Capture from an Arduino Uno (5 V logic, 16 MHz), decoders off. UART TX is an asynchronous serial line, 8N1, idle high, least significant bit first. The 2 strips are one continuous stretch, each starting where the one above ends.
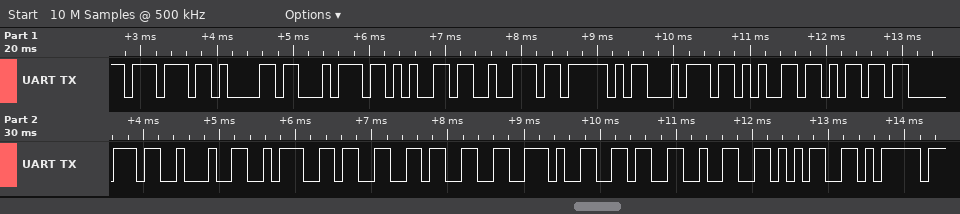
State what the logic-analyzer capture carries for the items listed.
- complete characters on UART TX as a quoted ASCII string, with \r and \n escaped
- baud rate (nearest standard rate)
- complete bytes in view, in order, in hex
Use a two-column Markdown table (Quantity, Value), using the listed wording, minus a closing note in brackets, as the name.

| Quantity | Value |
|---|---|
| complete characters on UART TX as a quoted ASCII string, with \r and \n escaped | "water_temp\":33.625}" |
| baud rate | 9600 baud |
| complete bytes in view, in order, in hex | 0x77 0x61 0x74 0x65 0x72 0x5F 0x74 0x65 0x6D 0x70 0x22 0x3A 0x33 0x33 0x2E 0x36 0x32 0x35 0x7D |
